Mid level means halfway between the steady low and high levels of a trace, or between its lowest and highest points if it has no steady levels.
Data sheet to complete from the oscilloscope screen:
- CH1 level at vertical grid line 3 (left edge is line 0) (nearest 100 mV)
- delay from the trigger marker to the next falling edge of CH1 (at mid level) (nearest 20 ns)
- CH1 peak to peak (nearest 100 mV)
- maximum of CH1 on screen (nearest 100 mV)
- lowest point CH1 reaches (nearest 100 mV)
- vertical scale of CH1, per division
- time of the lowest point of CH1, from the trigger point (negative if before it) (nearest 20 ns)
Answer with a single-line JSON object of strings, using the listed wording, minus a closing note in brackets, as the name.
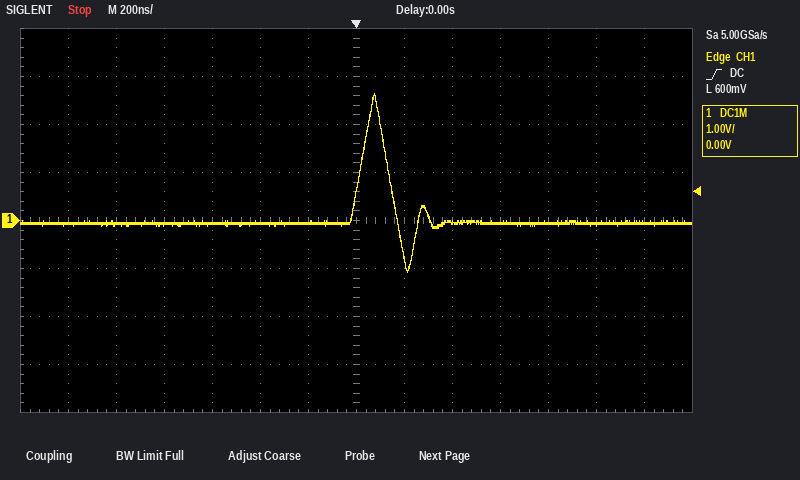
{"CH1 level at vertical grid line 3 (left edge is line 0)": "-100 mV", "delay from the trigger marker to the next falling edge of CH1 (at mid level)": "140 ns", "CH1 peak to peak": "3.7 V", "maximum of CH1 on screen": "2.6 V", "lowest point CH1 reaches": "-1.1 V", "vertical scale of CH1, per division": "1 V", "time of the lowest point of CH1, from the trigger point (negative if before it)": "+220 ns"}
